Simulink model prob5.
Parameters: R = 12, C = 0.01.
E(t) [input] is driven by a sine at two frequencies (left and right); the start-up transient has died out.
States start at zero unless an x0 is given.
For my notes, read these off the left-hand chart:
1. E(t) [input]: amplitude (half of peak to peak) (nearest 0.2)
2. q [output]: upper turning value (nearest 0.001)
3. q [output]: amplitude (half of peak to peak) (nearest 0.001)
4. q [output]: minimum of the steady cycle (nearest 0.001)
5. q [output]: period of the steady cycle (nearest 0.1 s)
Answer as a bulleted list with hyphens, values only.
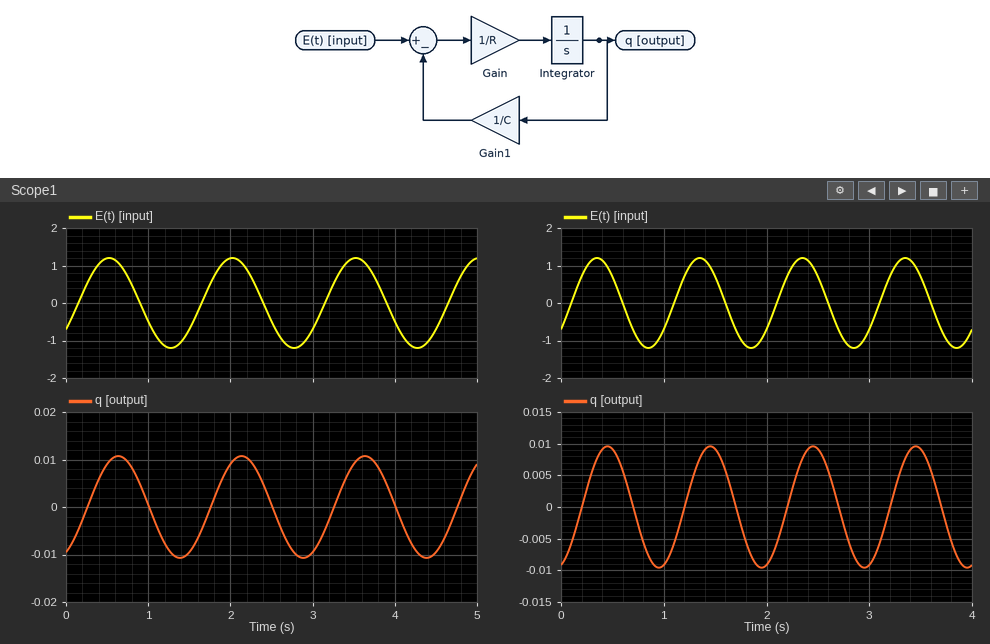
- 1.2
- 0.011
- 0.011
- -0.011
- 1.5 s
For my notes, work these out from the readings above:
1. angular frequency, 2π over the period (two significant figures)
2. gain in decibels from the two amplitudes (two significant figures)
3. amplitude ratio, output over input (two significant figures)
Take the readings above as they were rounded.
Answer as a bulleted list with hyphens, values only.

- 4.2 rad/s
- -41 dB
- 0.0092
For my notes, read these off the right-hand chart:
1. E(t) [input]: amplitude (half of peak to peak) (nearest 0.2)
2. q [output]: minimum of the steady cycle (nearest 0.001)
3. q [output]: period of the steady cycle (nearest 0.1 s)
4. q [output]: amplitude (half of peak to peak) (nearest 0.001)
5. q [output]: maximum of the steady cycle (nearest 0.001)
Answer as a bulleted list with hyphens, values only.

- 1.2
- -0.010
- 1.0 s
- 0.010
- 0.010
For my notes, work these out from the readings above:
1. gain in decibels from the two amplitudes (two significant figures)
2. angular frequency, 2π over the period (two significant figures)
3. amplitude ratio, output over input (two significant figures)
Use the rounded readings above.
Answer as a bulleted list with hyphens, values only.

- -42 dB
- 6.3 rad/s
- 0.0083
